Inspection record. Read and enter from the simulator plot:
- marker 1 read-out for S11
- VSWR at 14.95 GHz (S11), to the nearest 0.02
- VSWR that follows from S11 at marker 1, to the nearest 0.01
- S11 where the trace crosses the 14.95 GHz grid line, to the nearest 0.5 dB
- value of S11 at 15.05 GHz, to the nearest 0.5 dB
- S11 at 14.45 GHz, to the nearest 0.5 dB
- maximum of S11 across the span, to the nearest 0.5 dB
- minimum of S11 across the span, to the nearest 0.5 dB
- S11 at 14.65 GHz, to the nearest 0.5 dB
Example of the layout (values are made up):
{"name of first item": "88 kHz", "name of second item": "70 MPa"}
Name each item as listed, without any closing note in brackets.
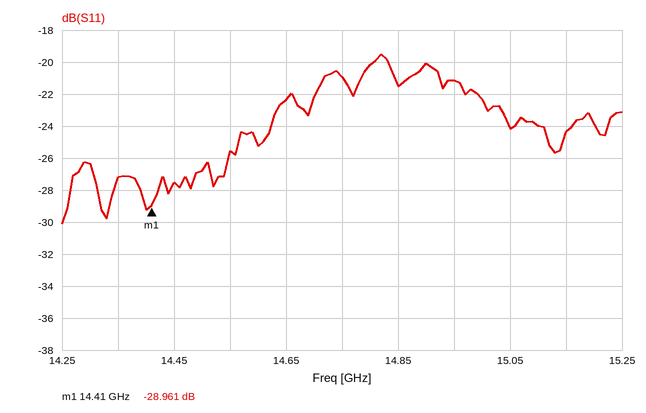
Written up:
{"marker 1 read-out for S11": "-28.961 dB", "VSWR at 14.95 GHz (S11), to the nearest 0.02": "1.20", "VSWR that follows from S11 at marker 1, to the nearest 0.01": "1.07", "S11 where the trace crosses the 14.95 GHz grid line, to the nearest 0.5 dB": "-21.0 dB", "value of S11 at 15.05 GHz, to the nearest 0.5 dB": "-24.0 dB", "S11 at 14.45 GHz, to the nearest 0.5 dB": "-27.5 dB", "maximum of S11 across the span, to the nearest 0.5 dB": "-19.5 dB", "minimum of S11 across the span, to the nearest 0.5 dB": "-30.0 dB", "S11 at 14.65 GHz, to the nearest 0.5 dB": "-22.5 dB"}
